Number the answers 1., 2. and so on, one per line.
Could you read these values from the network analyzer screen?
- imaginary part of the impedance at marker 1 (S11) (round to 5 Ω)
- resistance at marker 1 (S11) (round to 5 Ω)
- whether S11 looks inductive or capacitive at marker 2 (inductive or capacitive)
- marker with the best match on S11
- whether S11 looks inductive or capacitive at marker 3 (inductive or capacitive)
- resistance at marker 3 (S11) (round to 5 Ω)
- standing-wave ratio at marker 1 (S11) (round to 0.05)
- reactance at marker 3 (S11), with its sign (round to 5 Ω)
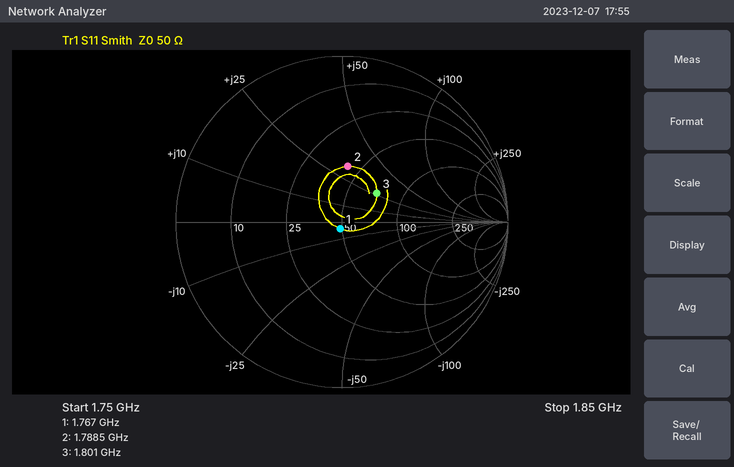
1. -5 Ω
2. 50 Ω
3. inductive
4. marker 1
5. inductive
6. 70 Ω
7. 1.10
8. +25 Ω
